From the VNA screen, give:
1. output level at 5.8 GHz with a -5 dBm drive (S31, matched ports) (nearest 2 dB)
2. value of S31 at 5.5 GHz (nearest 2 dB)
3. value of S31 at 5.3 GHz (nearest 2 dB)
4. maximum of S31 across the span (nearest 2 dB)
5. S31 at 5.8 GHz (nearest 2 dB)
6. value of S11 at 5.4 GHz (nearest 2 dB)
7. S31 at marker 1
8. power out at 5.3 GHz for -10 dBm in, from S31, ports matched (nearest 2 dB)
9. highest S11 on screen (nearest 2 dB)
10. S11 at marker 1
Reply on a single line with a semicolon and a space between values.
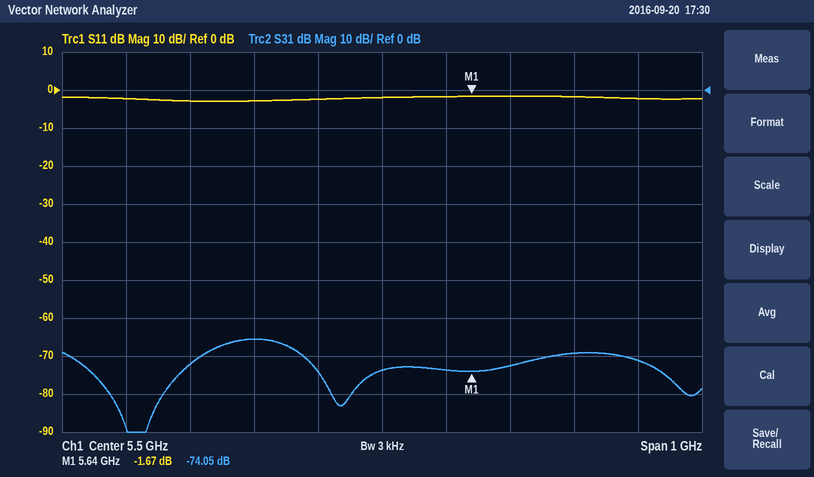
-74 dBm; -74 dB; -66 dB; -66 dB; -70 dB; -2 dB; -74.05 dB; -76 dBm; -2 dB; -1.67 dB
